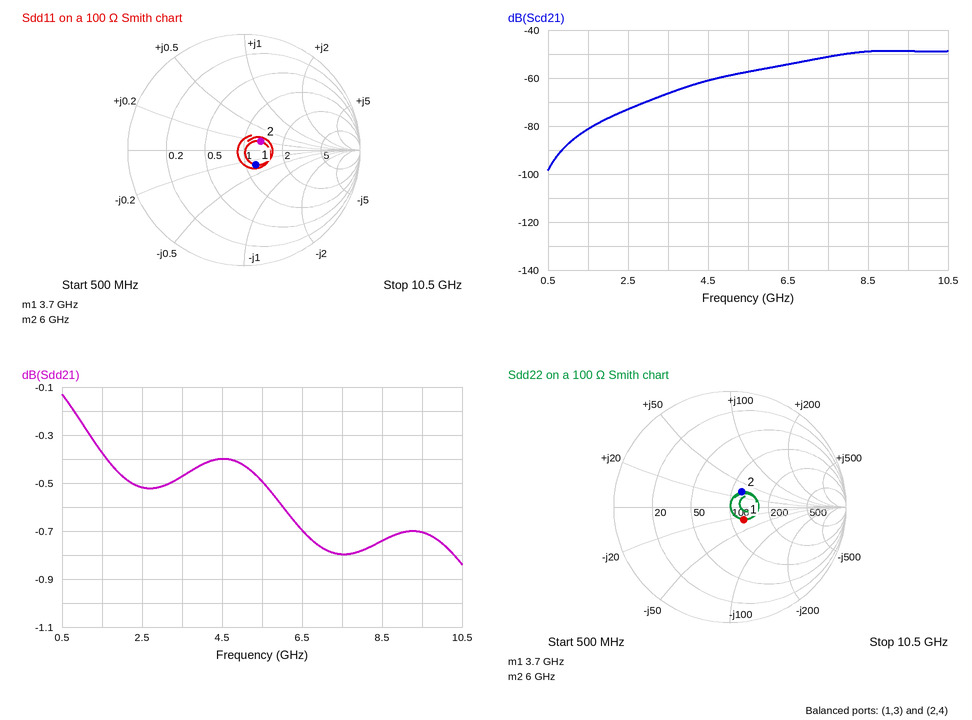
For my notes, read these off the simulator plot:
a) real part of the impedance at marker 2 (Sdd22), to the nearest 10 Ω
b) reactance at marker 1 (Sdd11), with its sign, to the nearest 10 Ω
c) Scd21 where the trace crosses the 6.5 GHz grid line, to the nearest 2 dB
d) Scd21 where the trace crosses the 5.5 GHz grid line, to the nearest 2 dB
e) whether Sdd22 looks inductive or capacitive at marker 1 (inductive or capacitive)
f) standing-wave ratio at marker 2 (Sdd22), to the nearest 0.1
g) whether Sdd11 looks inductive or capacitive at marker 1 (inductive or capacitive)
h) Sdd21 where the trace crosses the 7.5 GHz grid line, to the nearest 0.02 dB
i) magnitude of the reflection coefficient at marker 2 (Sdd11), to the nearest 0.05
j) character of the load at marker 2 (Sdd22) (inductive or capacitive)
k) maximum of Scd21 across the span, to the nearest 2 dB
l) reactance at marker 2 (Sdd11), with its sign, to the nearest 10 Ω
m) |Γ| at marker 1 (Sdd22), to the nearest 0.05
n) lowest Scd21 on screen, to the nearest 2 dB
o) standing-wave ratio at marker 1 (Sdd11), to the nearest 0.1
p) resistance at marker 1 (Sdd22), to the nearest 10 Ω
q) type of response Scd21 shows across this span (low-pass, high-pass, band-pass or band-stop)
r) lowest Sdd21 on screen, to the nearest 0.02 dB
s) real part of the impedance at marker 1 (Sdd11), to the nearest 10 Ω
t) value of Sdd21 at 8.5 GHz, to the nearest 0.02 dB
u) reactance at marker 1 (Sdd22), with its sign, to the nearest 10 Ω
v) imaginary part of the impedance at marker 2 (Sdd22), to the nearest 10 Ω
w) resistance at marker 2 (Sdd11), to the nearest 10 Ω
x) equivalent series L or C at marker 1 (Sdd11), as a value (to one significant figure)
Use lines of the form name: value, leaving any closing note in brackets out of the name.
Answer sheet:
real part of the impedance at marker 2 (Sdd22), to the nearest 10 Ω: 120 Ω
reactance at marker 1 (Sdd11), with its sign, to the nearest 10 Ω: -30 Ω
Scd21 where the trace crosses the 6.5 GHz grid line, to the nearest 2 dB: -54 dB
Scd21 where the trace crosses the 5.5 GHz grid line, to the nearest 2 dB: -58 dB
whether Sdd22 looks inductive or capacitive at marker 1: capacitive
standing-wave ratio at marker 2 (Sdd22), to the nearest 0.1: 1.4
whether Sdd11 looks inductive or capacitive at marker 1: capacitive
Sdd21 where the trace crosses the 7.5 GHz grid line, to the nearest 0.02 dB: -0.80 dB
magnitude of the reflection coefficient at marker 2 (Sdd11), to the nearest 0.05: 0.15
character of the load at marker 2 (Sdd22): inductive
maximum of Scd21 across the span, to the nearest 2 dB: -48 dB
reactance at marker 2 (Sdd11), with its sign, to the nearest 10 Ω: +20 Ω
|Γ| at marker 1 (Sdd22), to the nearest 0.05: 0.15
lowest Scd21 on screen, to the nearest 2 dB: -98 dB
standing-wave ratio at marker 1 (Sdd11), to the nearest 0.1: 1.4
resistance at marker 1 (Sdd22), to the nearest 10 Ω: 120 Ω
type of response Scd21 shows across this span: high-pass
lowest Sdd21 on screen, to the nearest 0.02 dB: -0.84 dB
real part of the impedance at marker 1 (Sdd11), to the nearest 10 Ω: 120 Ω
value of Sdd21 at 8.5 GHz, to the nearest 0.02 dB: -0.74 dB
reactance at marker 1 (Sdd22), with its sign, to the nearest 10 Ω: -30 Ω
imaginary part of the impedance at marker 2 (Sdd22), to the nearest 10 Ω: +30 Ω
resistance at marker 2 (Sdd11), to the nearest 10 Ω: 130 Ω
equivalent series L or C at marker 1 (Sdd11), as a value: 1 pF
